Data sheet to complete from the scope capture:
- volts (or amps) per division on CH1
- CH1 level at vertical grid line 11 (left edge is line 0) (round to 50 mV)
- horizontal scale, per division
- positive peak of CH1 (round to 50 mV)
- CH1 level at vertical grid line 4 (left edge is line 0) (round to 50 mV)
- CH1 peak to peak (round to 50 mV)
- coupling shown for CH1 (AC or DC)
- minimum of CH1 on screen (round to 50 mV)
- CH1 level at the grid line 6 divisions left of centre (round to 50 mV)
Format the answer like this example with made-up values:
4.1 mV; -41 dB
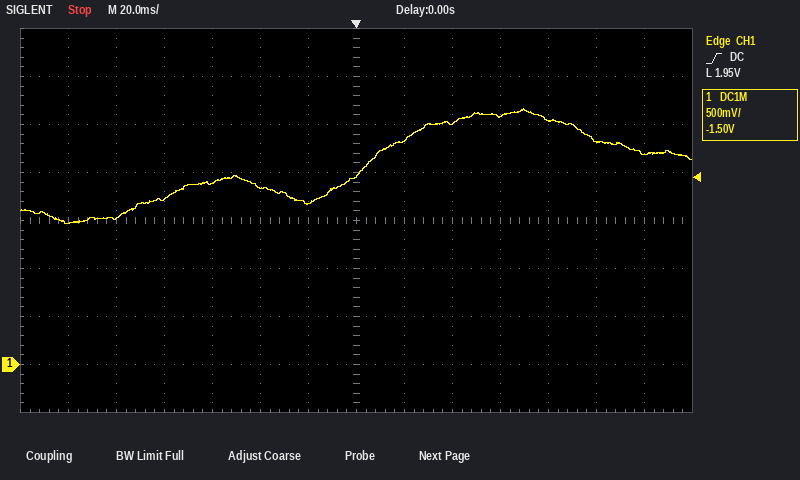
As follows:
500 mV; 2.55 V; 20 ms; 2.65 V; 1.90 V; 1.20 V; DC; 1.45 V; 1.45 V
